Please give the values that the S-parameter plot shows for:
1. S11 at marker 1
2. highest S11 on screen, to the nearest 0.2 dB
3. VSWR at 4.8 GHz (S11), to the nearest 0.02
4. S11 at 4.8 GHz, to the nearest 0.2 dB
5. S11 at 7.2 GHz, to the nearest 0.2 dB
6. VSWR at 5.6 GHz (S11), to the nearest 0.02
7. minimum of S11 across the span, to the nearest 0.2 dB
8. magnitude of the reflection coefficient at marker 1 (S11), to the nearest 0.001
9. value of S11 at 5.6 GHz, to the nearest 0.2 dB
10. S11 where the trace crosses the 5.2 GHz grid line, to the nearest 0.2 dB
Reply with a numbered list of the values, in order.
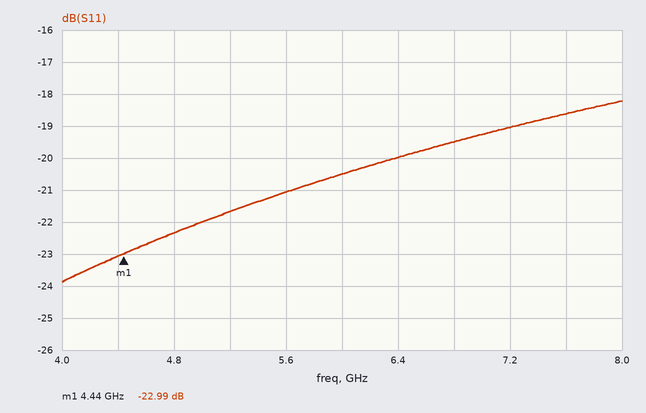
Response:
1. -22.99 dB
2. -18.2 dB
3. 1.16
4. -22.4 dB
5. -19.0 dB
6. 1.20
7. -23.8 dB
8. 0.071
9. -21.0 dB
10. -21.6 dB
